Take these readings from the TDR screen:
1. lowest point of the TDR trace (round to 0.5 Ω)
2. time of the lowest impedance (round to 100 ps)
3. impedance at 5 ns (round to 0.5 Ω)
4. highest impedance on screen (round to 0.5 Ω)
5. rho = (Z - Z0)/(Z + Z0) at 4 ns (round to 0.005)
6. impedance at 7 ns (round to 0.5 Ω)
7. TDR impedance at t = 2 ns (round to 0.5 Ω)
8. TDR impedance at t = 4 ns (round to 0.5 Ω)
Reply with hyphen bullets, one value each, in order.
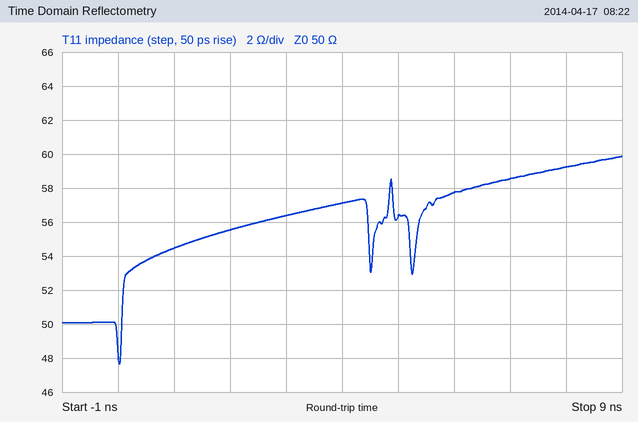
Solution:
- 47.5 Ω
- 0.0 ns
- 56.5 Ω
- 60.0 Ω
- +0.065
- 58.5 Ω
- 55.5 Ω
- 57.0 Ω
